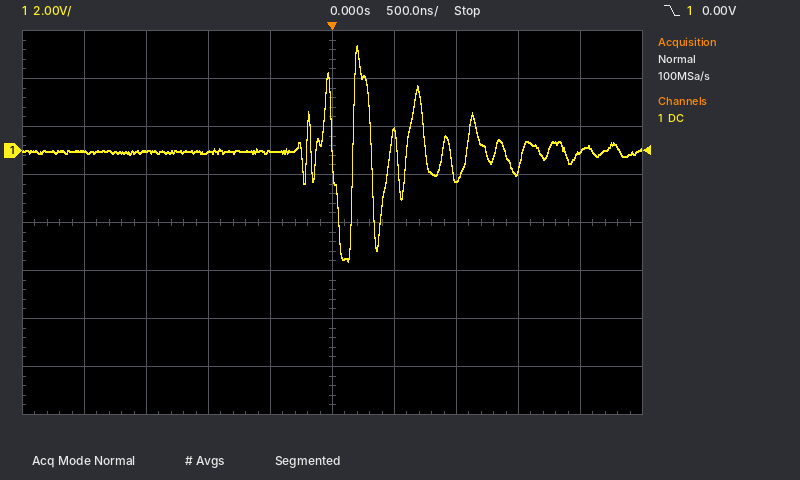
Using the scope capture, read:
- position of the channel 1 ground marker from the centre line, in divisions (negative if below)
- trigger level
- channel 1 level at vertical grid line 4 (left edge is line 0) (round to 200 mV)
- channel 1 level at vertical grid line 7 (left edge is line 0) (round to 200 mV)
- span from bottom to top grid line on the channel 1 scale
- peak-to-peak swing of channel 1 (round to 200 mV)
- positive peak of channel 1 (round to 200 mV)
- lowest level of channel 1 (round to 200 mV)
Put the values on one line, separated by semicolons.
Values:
+1.5 div; 0.00 V; 0.0 V; -1.2 V; 16 V; 9.0 V; 4.4 V; -4.6 V
